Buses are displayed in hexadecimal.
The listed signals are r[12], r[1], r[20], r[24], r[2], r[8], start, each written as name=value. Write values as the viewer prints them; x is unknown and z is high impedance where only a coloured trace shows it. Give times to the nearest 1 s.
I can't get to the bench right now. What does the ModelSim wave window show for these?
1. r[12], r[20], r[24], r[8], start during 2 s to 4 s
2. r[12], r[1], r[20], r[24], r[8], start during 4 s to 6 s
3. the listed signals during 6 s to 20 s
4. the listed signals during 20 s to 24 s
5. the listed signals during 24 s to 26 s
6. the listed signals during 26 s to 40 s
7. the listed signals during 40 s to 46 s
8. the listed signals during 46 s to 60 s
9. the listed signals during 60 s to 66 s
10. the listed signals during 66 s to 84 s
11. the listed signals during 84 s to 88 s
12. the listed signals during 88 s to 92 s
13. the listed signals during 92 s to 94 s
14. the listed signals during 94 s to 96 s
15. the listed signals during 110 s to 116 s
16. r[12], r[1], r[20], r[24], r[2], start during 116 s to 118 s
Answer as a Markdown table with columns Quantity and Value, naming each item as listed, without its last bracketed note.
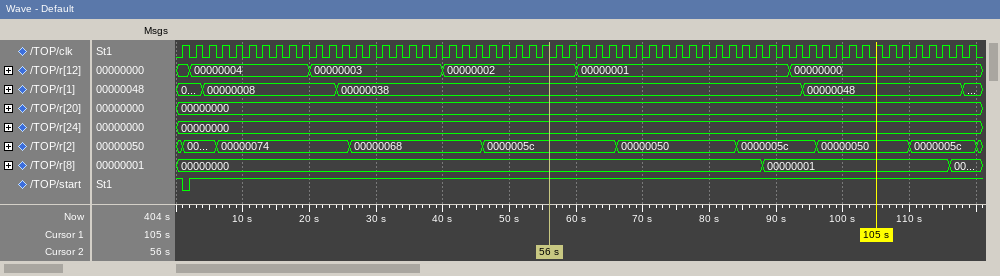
| Quantity | Value |
|---|---|
| r[12], r[20], r[24], r[8], start during 2 s to 4 s | r[12]=00000004, r[20]=00000000, r[24]=00000000, r[8]=00000000, start=1 |
| r[12], r[1], r[20], r[24], r[8], start during 4 s to 6 s | r[12]=00000004, r[1]=00000008, r[20]=00000000, r[24]=00000000, r[8]=00000000, start=1 |
| the listed signals during 6 s to 20 s | r[12]=00000004, r[1]=00000008, r[20]=00000000, r[24]=00000000, r[2]=00000074, r[8]=00000000, start=1 |
| the listed signals during 20 s to 24 s | r[12]=00000003, r[1]=00000008, r[20]=00000000, r[24]=00000000, r[2]=00000074, r[8]=00000000, start=1 |
| the listed signals during 24 s to 26 s | r[12]=00000003, r[1]=00000038, r[20]=00000000, r[24]=00000000, r[2]=00000074, r[8]=00000000, start=1 |
| the listed signals during 26 s to 40 s | r[12]=00000003, r[1]=00000038, r[20]=00000000, r[24]=00000000, r[2]=00000068, r[8]=00000000, start=1 |
| the listed signals during 40 s to 46 s | r[12]=00000002, r[1]=00000038, r[20]=00000000, r[24]=00000000, r[2]=00000068, r[8]=00000000, start=1 |
| the listed signals during 46 s to 60 s | r[12]=00000002, r[1]=00000038, r[20]=00000000, r[24]=00000000, r[2]=0000005c, r[8]=00000000, start=1 |
| the listed signals during 60 s to 66 s | r[12]=00000001, r[1]=00000038, r[20]=00000000, r[24]=00000000, r[2]=0000005c, r[8]=00000000, start=1 |
| the listed signals during 66 s to 84 s | r[12]=00000001, r[1]=00000038, r[20]=00000000, r[24]=00000000, r[2]=00000050, r[8]=00000000, start=1 |
| the listed signals during 84 s to 88 s | r[12]=00000001, r[1]=00000038, r[20]=00000000, r[24]=00000000, r[2]=0000005c, r[8]=00000000, start=1 |
| the listed signals during 88 s to 92 s | r[12]=00000001, r[1]=00000038, r[20]=00000000, r[24]=00000000, r[2]=0000005c, r[8]=00000001, start=1 |
| the listed signals during 92 s to 94 s | r[12]=00000000, r[1]=00000038, r[20]=00000000, r[24]=00000000, r[2]=0000005c, r[8]=00000001, start=1 |
| the listed signals during 94 s to 96 s | r[12]=00000000, r[1]=00000048, r[20]=00000000, r[24]=00000000, r[2]=0000005c, r[8]=00000001, start=1 |
| the listed signals during 110 s to 116 s | r[12]=00000000, r[1]=00000048, r[20]=00000000, r[24]=00000000, r[2]=0000005c, r[8]=00000001, start=1 |
| r[12], r[1], r[20], r[24], r[2], start during 116 s to 118 s | r[12]=00000000, r[1]=00000048, r[20]=00000000, r[24]=00000000, r[2]=0000005c, start=1 |
